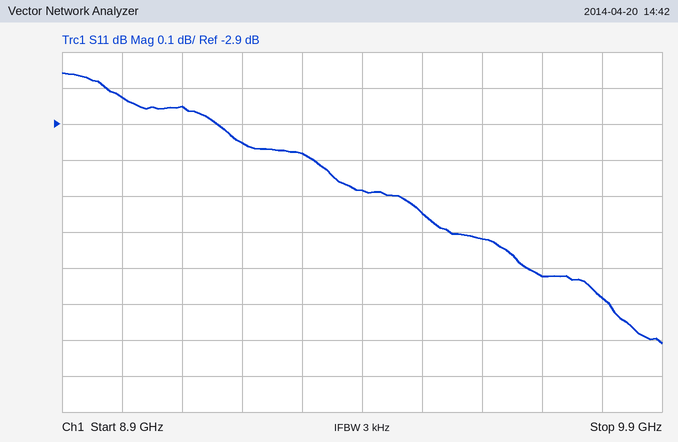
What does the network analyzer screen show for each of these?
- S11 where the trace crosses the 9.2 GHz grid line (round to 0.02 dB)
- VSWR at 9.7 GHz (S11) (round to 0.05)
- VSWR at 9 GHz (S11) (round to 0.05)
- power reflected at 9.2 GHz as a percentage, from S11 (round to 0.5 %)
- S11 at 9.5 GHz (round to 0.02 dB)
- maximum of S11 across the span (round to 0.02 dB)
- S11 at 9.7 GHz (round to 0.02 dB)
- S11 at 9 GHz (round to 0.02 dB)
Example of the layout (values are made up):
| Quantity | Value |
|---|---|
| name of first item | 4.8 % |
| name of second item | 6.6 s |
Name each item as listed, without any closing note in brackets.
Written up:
| Quantity | Value |
|---|---|
| S11 where the trace crosses the 9.2 GHz grid line | -2.96 dB |
| VSWR at 9.7 GHz (S11) | 5.30 |
| VSWR at 9 GHz (S11) | 6.20 |
| power reflected at 9.2 GHz as a percentage, from S11 | 50.5 % |
| S11 at 9.5 GHz | -3.14 dB |
| maximum of S11 across the span | -2.76 dB |
| S11 at 9.7 GHz | -3.32 dB |
| S11 at 9 GHz | -2.82 dB |
